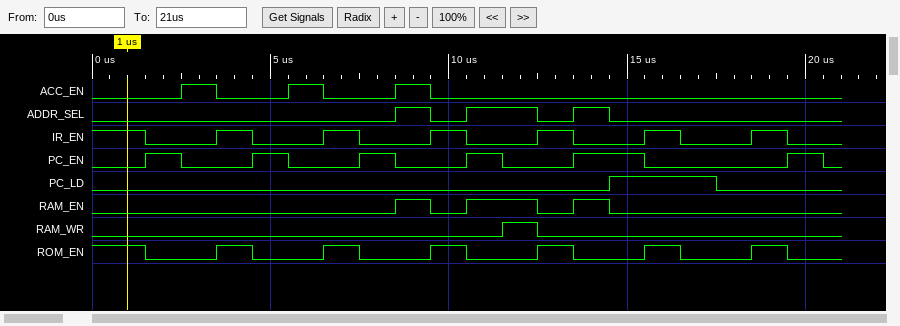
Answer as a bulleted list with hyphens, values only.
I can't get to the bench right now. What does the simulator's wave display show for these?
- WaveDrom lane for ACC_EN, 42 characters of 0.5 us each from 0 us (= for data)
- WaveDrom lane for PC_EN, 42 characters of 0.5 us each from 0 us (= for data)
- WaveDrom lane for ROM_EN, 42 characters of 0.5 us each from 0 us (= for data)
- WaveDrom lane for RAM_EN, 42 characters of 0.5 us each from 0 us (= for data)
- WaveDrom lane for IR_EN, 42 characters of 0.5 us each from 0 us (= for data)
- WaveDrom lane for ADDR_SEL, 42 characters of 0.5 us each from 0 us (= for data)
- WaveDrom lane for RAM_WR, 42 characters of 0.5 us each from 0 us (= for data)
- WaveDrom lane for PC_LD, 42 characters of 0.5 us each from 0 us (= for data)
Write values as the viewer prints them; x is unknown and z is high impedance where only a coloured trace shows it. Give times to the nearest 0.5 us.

- {name: 'ACC_EN', wave: '0....1.0...1.0...1.0......................'}
- {name: 'PC_EN', wave: '0..1.0...1.0...1.0...1.0...1...0.......1.0'}
- {name: 'ROM_EN', wave: '1..0...1.0...1.0...1.0...1.0...1.0...1.0..'}
- {name: 'RAM_EN', wave: '0................1.0.1...0.1.0............'}
- {name: 'IR_EN', wave: '1..0...1.0...1.0...1.0...1.0...1.0...1.0..'}
- {name: 'ADDR_SEL', wave: '0................1.0.1...0.1.0............'}
- {name: 'RAM_WR', wave: '0......................1.0................'}
- {name: 'PC_LD', wave: '0............................1.....0......'}
